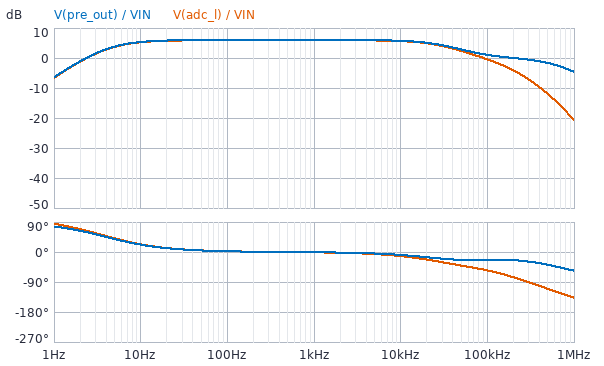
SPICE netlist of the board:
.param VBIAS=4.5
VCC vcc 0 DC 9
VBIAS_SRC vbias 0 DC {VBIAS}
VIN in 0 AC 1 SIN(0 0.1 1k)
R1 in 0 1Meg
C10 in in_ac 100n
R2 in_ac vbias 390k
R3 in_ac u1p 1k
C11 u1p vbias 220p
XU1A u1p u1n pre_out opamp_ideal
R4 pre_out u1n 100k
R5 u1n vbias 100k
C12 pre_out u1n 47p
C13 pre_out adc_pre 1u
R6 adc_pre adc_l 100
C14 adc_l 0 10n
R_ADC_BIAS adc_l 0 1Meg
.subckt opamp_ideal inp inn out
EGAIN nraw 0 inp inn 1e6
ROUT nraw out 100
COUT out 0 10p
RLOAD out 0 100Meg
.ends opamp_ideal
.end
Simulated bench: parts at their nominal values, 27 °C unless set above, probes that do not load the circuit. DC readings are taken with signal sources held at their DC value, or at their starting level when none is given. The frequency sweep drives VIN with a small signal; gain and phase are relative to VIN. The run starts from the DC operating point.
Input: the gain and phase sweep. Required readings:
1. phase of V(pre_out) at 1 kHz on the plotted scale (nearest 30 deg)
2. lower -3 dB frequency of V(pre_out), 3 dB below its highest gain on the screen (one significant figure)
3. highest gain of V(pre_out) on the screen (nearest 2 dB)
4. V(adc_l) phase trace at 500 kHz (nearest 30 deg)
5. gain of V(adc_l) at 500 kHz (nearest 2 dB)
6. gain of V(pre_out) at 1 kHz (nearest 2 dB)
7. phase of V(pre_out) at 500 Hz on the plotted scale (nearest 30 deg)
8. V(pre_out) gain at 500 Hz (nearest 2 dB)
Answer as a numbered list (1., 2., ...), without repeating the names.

1. 0 deg
2. 4 Hz
3. 6 dB
4. -120 deg
5. -12 dB
6. 6 dB
7. 0 deg
8. 6 dB
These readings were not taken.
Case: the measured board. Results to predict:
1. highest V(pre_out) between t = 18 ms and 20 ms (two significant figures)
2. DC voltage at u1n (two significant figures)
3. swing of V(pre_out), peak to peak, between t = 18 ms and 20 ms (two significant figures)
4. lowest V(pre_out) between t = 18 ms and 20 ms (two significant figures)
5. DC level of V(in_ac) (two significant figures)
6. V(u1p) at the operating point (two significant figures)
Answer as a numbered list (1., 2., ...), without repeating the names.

1. 4.7 V
2. 4.5 V
3. 400 mV
4. 4.3 V
5. 4.5 V
6. 4.5 V
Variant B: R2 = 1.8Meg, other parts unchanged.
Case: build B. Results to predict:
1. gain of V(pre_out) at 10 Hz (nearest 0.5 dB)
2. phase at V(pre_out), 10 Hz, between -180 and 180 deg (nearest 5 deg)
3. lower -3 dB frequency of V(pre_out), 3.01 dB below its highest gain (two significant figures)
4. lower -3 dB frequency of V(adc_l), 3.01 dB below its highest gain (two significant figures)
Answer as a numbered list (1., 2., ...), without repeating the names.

1. 6.0 dB
2. 5 deg
3. 880 mHz
4. 910 mHz
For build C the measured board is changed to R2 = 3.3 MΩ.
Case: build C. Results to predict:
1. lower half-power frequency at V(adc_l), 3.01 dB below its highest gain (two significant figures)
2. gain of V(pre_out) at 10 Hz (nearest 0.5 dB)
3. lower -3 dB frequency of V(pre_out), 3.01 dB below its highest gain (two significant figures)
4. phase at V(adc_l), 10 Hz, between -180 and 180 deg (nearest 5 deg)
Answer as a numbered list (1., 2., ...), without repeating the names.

1. 530 mHz
2. 6.0 dB
3. 480 mHz
4. 5 deg
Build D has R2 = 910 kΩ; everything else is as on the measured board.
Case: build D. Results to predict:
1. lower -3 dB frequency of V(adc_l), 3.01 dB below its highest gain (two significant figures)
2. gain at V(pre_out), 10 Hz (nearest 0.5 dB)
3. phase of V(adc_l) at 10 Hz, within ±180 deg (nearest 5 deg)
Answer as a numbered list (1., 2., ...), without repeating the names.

1. 1.8 Hz
2. 6.0 dB
3. 10 deg
